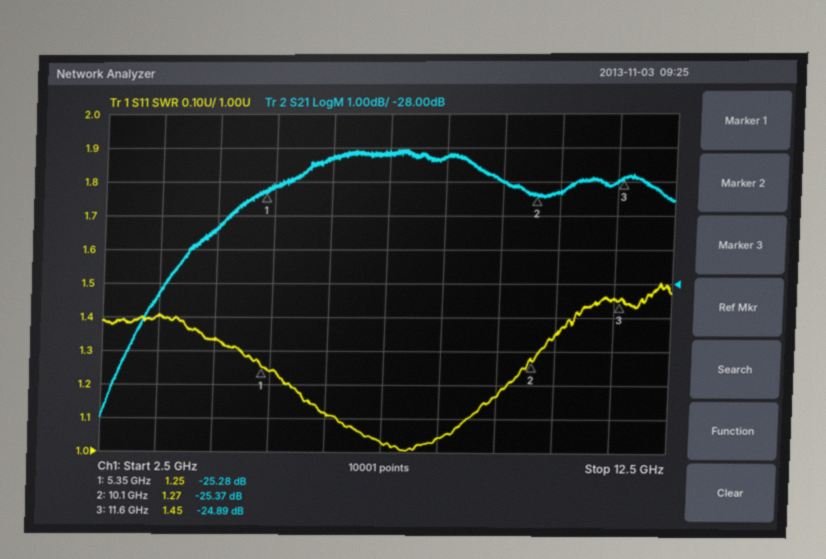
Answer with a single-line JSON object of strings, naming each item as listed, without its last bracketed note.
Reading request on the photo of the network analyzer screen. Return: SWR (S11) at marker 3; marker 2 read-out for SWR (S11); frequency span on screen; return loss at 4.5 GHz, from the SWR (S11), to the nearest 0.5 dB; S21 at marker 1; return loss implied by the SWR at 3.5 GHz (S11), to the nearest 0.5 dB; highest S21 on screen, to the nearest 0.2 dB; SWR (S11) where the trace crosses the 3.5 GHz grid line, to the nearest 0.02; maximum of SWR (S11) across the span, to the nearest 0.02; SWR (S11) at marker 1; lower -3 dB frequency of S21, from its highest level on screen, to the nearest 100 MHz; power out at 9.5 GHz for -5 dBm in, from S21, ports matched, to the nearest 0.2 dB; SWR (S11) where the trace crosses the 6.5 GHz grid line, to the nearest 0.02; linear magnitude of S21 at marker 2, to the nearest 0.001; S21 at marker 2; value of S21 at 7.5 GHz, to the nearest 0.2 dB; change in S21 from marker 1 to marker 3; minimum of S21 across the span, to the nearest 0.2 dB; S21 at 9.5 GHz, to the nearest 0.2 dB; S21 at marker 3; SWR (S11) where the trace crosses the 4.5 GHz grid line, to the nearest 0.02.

{"SWR (S11) at marker 3": "1.45", "marker 2 read-out for SWR": "1.27", "frequency span on screen": "10 GHz", "return loss at 4.5 GHz, from the SWR (S11), to the nearest 0.5 dB": "17.0 dB", "S21 at marker 1": "-25.28 dB", "return loss implied by the SWR at 3.5 GHz (S11), to the nearest 0.5 dB": "15.5 dB", "highest S21 on screen, to the nearest 0.2 dB": "-24.0 dB", "SWR (S11) where the trace crosses the 3.5 GHz grid line, to the nearest 0.02": "1.40", "maximum of SWR (S11) across the span, to the nearest 0.02": "1.50", "SWR (S11) at marker 1": "1.25", "lower -3 dB frequency of S21, from its highest level on screen, to the nearest 100 MHz": "4.0 GHz", "power out at 9.5 GHz for -5 dBm in, from S21, ports matched, to the nearest 0.2 dB": "-30.0 dBm", "SWR (S11) where the trace crosses the 6.5 GHz grid line, to the nearest 0.02": "1.12", "linear magnitude of S21 at marker 2, to the nearest 0.001": "0.054", "S21 at marker 2": "-25.37 dB", "value of S21 at 7.5 GHz, to the nearest 0.2 dB": "-24.2 dB", "change in S21 from marker 1 to marker 3": "0.39 dB", "minimum of S21 across the span, to the nearest 0.2 dB": "-32.0 dB", "S21 at 9.5 GHz, to the nearest 0.2 dB": "-25.0 dB", "S21 at marker 3": "-24.89 dB", "SWR (S11) where the trace crosses the 4.5 GHz grid line, to the nearest 0.02": "1.34"}
